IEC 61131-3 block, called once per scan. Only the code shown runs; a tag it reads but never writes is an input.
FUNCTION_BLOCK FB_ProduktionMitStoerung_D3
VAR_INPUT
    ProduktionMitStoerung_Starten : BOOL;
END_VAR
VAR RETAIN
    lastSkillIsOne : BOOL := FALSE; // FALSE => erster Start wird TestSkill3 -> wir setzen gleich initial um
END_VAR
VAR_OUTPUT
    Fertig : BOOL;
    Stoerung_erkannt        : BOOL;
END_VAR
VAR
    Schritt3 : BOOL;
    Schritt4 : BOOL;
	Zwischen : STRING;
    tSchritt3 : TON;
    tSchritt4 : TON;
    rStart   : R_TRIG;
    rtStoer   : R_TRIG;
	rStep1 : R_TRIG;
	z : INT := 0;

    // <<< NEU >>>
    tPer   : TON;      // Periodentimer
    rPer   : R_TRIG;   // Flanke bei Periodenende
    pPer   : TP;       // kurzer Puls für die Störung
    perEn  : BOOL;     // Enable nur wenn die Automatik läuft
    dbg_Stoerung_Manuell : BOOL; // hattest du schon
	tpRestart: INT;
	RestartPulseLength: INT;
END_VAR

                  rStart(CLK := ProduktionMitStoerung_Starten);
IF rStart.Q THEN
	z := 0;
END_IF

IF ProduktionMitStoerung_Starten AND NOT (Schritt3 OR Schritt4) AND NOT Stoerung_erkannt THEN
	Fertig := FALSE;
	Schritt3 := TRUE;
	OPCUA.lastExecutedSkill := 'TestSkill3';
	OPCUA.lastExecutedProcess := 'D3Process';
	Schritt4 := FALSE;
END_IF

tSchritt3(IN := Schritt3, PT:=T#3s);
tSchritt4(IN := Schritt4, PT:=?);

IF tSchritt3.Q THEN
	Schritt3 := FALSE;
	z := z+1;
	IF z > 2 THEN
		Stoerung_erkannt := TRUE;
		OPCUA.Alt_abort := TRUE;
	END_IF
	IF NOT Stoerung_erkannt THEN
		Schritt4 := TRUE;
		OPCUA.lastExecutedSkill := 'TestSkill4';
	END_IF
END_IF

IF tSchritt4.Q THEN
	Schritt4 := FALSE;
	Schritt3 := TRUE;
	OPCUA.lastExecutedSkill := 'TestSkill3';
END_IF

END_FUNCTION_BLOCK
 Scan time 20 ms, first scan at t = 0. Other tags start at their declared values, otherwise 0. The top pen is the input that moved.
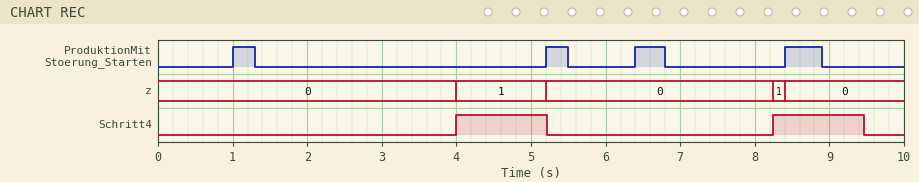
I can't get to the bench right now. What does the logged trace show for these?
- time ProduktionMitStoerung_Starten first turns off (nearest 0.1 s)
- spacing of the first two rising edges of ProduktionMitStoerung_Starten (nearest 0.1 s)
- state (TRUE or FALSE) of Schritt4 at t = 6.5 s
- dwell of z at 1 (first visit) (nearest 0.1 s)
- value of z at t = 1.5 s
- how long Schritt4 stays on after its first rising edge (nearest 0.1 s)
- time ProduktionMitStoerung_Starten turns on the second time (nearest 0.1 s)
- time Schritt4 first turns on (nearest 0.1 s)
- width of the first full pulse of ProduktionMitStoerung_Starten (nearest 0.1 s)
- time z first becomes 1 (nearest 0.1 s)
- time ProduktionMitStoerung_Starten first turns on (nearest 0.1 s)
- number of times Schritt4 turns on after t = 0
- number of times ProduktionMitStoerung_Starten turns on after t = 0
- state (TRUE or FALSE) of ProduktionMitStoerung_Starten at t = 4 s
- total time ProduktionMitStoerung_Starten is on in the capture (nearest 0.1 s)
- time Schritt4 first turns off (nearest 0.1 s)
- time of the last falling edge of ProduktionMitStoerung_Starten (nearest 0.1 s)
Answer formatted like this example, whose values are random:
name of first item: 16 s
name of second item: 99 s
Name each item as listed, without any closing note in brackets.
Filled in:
time ProduktionMitStoerung_Starten first turns off: 1.3 s
spacing of the first two rising edges of ProduktionMitStoerung_Starten: 4.2 s
state (TRUE or FALSE) of Schritt4 at t = 6.5 s: FALSE
dwell of z at 1 (first visit): 1.2 s
value of z at t = 1.5 s: 0
how long Schritt4 stays on after its first rising edge: 1.2 s
time ProduktionMitStoerung_Starten turns on the second time: 5.2 s
time Schritt4 first turns on: 4.0 s
width of the first full pulse of ProduktionMitStoerung_Starten: 0.3 s
time z first becomes 1: 4.0 s
time ProduktionMitStoerung_Starten first turns on: 1.0 s
number of times Schritt4 turns on after t = 0: 2
number of times ProduktionMitStoerung_Starten turns on after t = 0: 4
state (TRUE or FALSE) of ProduktionMitStoerung_Starten at t = 4 s: FALSE
total time ProduktionMitStoerung_Starten is on in the capture: 1.5 s
time Schritt4 first turns off: 5.2 s
time of the last falling edge of ProduktionMitStoerung_Starten: 8.9 s
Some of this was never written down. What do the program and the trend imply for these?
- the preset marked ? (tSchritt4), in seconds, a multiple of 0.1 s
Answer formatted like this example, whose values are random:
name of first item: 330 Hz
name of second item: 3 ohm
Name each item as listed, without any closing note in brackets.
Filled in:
the preset marked ? (tSchritt4), in seconds, a multiple of 0.1 s: 1.2 s
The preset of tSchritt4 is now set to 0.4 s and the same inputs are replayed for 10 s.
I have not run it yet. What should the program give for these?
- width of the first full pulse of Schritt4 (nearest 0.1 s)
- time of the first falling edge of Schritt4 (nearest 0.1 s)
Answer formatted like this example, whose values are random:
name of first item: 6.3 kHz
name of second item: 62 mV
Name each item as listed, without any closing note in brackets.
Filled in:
width of the first full pulse of Schritt4: 0.4 s
time of the first falling edge of Schritt4: 4.4 s
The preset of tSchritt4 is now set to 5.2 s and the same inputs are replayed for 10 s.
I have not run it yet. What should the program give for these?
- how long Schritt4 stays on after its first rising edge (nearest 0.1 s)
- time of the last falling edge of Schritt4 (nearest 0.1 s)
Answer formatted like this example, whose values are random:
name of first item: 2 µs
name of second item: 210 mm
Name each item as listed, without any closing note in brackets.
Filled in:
how long Schritt4 stays on after its first rising edge: 5.2 s
time of the last falling edge of Schritt4: 9.2 s
